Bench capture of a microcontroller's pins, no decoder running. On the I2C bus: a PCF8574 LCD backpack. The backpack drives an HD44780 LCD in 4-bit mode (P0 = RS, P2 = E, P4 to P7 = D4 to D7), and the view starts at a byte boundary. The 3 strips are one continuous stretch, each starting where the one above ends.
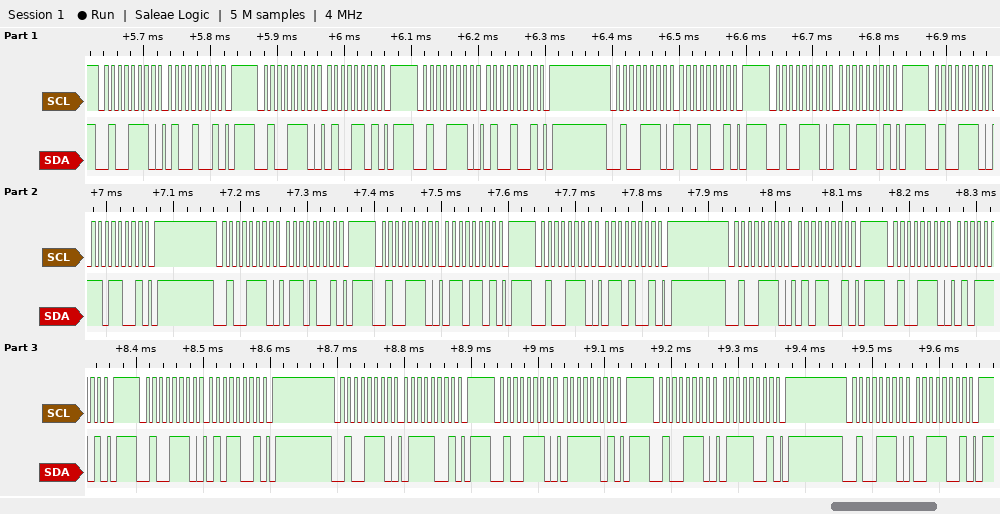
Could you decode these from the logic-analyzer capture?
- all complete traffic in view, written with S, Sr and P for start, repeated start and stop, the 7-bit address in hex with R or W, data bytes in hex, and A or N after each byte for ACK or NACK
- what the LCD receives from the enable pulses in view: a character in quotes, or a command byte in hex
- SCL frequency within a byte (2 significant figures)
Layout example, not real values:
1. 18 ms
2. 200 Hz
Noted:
1. S 27W A 49 A P S 27W A 4D A P S 27W A 49 A P S 27W A D9 A P S 27W A DD A P S 27W A D9 A P S 27W A 69 A P S 27W A 6D A P S 27W A 69 A P S 27W A 59 A P S 27W A 5D A P S 27W A 59 A P S 27W A 79 A P S 27W A 7D A P S 27W A 79 A P S 27W A 39 A P
2. 'M' 'e'
3. 100 kHz
